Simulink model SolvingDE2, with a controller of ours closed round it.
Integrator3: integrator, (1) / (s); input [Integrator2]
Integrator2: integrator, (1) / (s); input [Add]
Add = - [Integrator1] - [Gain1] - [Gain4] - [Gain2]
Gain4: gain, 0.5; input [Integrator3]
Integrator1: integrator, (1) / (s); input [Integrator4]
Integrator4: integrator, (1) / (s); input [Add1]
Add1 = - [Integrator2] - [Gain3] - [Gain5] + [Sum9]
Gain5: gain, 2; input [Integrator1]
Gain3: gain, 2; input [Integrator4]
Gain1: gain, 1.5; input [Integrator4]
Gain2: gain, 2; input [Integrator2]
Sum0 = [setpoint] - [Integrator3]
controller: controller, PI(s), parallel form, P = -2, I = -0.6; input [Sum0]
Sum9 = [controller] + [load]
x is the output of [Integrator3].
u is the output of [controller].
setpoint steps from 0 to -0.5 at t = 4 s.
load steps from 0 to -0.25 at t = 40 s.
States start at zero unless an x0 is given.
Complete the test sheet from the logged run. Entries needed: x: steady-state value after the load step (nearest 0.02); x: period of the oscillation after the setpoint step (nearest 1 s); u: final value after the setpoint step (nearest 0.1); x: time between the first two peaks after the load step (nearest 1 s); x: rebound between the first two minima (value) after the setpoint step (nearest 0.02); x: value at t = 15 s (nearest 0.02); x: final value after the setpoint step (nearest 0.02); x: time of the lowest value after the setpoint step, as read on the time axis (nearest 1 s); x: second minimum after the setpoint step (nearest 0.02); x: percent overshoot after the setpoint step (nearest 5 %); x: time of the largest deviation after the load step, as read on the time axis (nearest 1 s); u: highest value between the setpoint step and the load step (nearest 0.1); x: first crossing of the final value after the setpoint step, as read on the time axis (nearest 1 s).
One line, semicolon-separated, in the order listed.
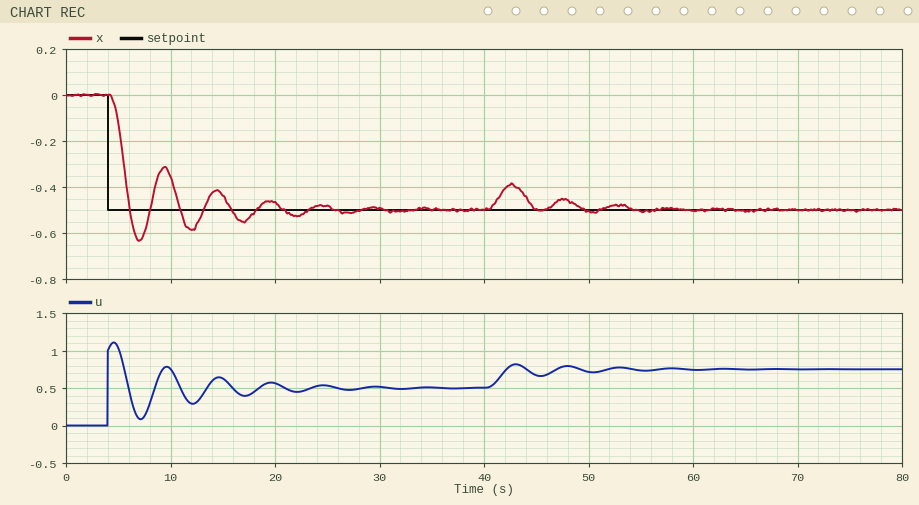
-0.50; 5 s; 0.5; 5 s; -0.32; -0.44; -0.50; 7 s; -0.58; 25 %; 43 s; 1.1; 6 s
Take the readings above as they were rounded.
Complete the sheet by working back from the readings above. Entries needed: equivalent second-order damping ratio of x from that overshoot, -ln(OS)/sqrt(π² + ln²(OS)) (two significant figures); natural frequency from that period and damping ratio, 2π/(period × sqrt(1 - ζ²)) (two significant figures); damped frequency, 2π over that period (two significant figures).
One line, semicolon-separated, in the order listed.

0.40; 1.4 rad/s; 1.3 rad/s
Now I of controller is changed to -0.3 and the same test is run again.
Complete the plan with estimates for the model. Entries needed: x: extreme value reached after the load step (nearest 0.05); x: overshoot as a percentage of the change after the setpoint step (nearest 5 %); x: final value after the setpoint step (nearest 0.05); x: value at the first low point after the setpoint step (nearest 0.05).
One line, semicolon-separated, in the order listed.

-0.40; 10 %; -0.50; -0.55
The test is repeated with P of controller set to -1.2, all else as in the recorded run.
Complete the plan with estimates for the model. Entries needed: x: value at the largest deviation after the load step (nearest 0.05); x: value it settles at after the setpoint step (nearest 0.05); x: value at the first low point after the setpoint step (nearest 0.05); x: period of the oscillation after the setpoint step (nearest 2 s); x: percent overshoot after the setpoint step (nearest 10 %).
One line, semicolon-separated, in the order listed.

-0.35; -0.50; -0.60; 6 s; 20 %
